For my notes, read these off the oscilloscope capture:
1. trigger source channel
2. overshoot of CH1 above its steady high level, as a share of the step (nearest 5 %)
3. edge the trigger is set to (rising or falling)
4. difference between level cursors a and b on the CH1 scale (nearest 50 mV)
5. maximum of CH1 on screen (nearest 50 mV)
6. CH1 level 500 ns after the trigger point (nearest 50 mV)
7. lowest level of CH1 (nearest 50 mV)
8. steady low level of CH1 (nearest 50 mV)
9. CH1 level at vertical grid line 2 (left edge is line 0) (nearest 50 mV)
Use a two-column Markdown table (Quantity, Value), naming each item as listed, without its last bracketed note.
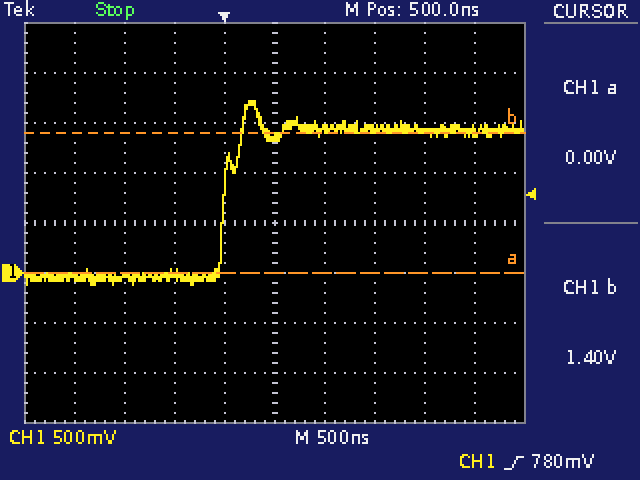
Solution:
| Quantity | Value |
|---|---|
| trigger source channel | CH1 |
| overshoot of CH1 above its steady high level, as a share of the step | 20 % |
| edge the trigger is set to | rising |
| difference between level cursors a and b on the CH1 scale | 1.40 V |
| maximum of CH1 on screen | 1.70 V |
| CH1 level 500 ns after the trigger point | 1.35 V |
| lowest level of CH1 | -100 mV |
| steady low level of CH1 | -50 mV |
| CH1 level at vertical grid line 2 (left edge is line 0) | -50 mV |
